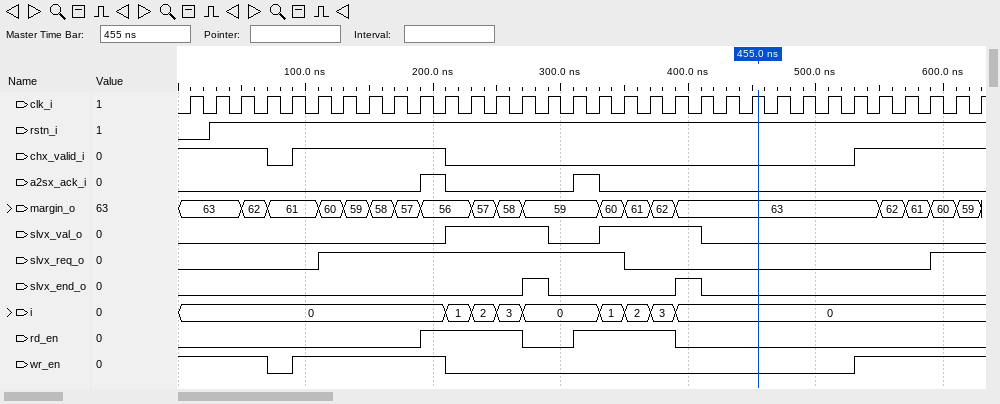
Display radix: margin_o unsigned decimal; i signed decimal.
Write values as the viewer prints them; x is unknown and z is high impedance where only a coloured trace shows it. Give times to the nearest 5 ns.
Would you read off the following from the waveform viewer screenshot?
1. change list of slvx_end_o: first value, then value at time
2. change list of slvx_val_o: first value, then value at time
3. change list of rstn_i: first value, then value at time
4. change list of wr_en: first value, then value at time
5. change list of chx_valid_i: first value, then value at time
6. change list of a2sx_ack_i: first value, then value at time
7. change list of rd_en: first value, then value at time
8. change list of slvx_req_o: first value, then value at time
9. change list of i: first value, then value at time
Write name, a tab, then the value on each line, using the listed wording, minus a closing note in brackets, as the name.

change list of slvx_end_o: first value, then value at time	0, 1 at 270 ns, 0 at 290 ns, 1 at 390 ns, 0 at 410 ns
change list of slvx_val_o: first value, then value at time	0, 1 at 210 ns, 0 at 290 ns, 1 at 330 ns, 0 at 410 ns
change list of rstn_i: first value, then value at time	0, 1 at 25 ns
change list of wr_en: first value, then value at time	1, 0 at 70 ns, 1 at 90 ns, 0 at 210 ns, 1 at 530 ns
change list of chx_valid_i: first value, then value at time	1, 0 at 70 ns, 1 at 90 ns, 0 at 210 ns, 1 at 530 ns
change list of a2sx_ack_i: first value, then value at time	0, 1 at 190 ns, 0 at 210 ns, 1 at 310 ns, 0 at 330 ns
change list of rd_en: first value, then value at time	0, 1 at 190 ns, 0 at 270 ns, 1 at 310 ns, 0 at 390 ns
change list of slvx_req_o: first value, then value at time	0, 1 at 110 ns, 0 at 350 ns, 1 at 590 ns
change list of i: first value, then value at time	0, 1 at 210 ns, 2 at 230 ns, 3 at 250 ns, 0 at 270 ns, 1 at 330 ns, 2 at 350 ns, 3 at 370 ns, 0 at 390 ns
